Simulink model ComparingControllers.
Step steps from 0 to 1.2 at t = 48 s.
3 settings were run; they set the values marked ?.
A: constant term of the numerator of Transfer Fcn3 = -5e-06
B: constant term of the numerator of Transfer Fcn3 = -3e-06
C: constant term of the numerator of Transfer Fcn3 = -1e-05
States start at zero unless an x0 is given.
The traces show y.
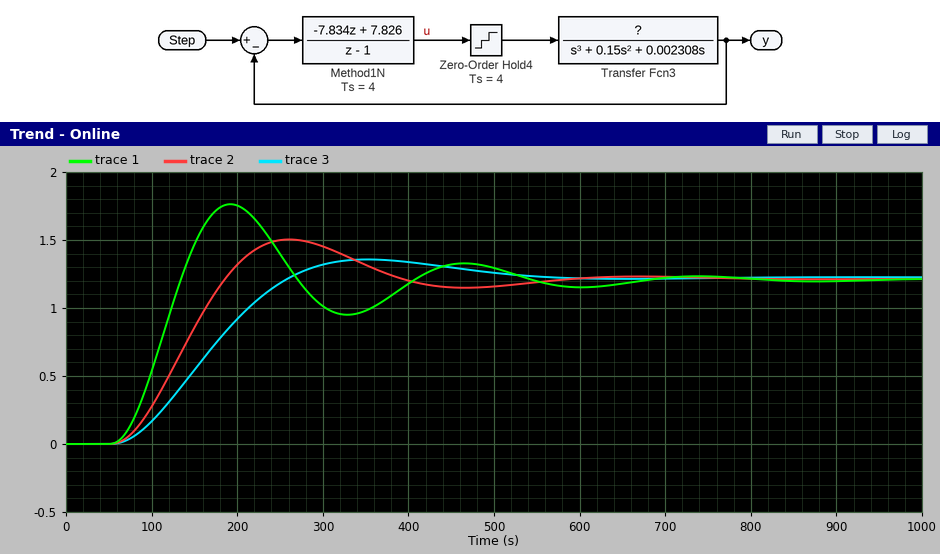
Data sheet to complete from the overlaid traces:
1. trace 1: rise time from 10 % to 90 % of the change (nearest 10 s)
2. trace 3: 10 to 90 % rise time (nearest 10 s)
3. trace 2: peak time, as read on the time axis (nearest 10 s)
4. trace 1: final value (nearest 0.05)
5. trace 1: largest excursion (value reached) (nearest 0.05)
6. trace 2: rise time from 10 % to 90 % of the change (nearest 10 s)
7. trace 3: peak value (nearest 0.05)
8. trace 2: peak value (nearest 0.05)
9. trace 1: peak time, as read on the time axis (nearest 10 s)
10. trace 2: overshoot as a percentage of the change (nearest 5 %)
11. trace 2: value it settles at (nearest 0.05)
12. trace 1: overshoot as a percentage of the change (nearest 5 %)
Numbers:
50 s
140 s
260 s
1.20
1.75
90 s
1.35
1.50
190 s
25 %
1.20
45 %
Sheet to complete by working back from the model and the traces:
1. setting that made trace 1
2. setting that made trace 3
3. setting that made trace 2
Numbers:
C
B
A
